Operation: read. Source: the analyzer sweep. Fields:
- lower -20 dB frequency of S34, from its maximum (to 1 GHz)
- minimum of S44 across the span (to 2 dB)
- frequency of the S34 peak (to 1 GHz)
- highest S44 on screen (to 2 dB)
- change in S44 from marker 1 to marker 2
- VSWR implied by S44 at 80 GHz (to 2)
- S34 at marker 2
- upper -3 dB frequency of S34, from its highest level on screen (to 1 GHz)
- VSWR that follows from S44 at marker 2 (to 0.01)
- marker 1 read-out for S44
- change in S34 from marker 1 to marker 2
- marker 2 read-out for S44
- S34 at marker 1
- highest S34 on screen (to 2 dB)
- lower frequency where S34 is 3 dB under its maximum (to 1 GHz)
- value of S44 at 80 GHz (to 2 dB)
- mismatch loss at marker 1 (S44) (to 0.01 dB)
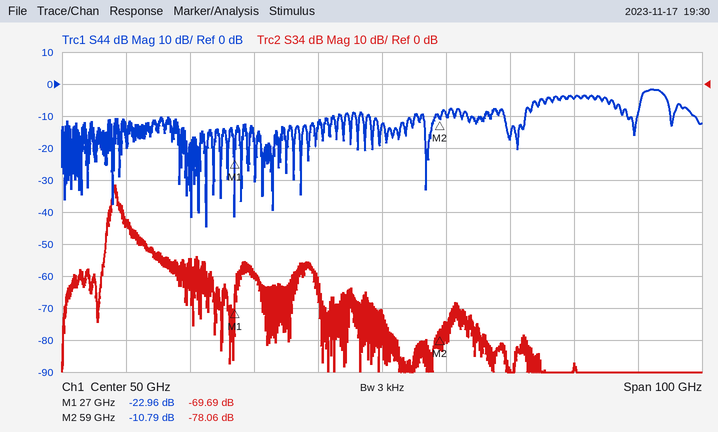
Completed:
7 GHz
-44 dB
8 GHz
-2 dB
12.17 dB
4
-78.06 dB
8 GHz
1.81
-22.96 dB
-8.37 dB
-10.79 dB
-69.69 dB
-32 dB
8 GHz
-4 dB
0.02 dB
